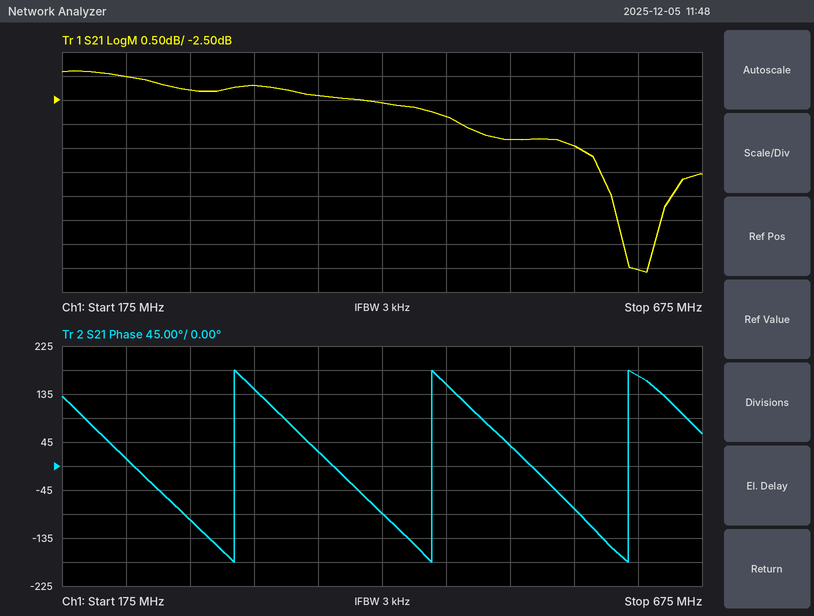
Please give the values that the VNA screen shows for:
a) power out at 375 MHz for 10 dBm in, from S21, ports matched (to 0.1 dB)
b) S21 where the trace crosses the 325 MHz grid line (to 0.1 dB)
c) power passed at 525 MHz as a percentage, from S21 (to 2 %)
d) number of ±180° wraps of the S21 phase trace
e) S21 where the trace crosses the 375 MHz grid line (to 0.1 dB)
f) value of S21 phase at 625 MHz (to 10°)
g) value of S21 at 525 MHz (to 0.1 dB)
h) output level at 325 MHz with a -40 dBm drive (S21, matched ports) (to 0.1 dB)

7.6 dBm
-2.2 dB
46 %
3
-2.4 dB
170°
-3.3 dB
-42.2 dBm
